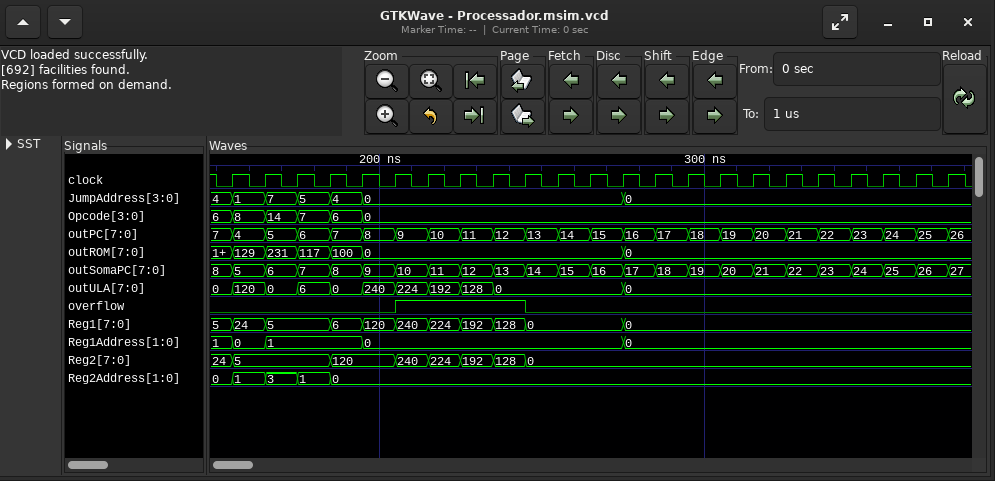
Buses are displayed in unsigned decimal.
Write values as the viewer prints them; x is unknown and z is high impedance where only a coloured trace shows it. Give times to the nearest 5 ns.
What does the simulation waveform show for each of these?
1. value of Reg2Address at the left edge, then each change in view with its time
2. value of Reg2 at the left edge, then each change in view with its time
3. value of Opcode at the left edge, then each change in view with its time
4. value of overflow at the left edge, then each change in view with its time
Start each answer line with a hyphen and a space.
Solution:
- 0, 1 at 155 ns, 3 at 165 ns, 1 at 175 ns, 0 at 185 ns
- 24, 5 at 155 ns, 120 at 185 ns, 240 at 205 ns, 224 at 215 ns, 192 at 225 ns, 128 at 235 ns, 0 at 245 ns
- 6, 8 at 155 ns, 14 at 165 ns, 7 at 175 ns, 6 at 185 ns, 0 at 195 ns
- 0, 1 at 205 ns, 0 at 245 ns
